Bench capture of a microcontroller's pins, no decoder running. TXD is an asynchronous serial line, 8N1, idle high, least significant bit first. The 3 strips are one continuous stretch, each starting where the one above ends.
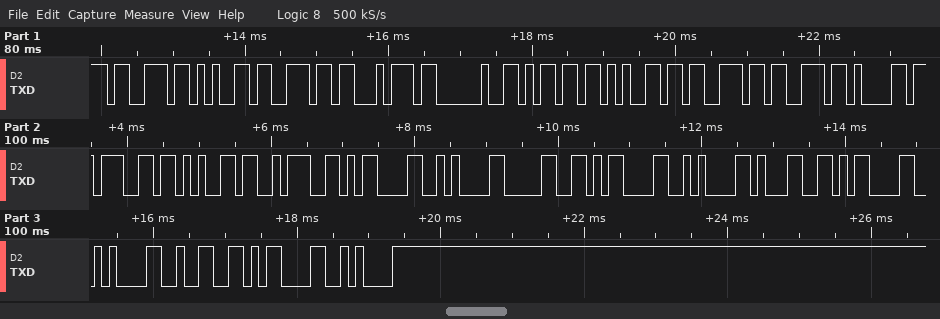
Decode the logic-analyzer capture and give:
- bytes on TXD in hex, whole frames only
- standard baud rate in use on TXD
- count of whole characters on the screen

73 65 6E 74 20 6D 65 73 73 61 67 65 3A 0D 0A 30 0D 0A 31 0D 0A 32 0D 0A
9600 baud
24
